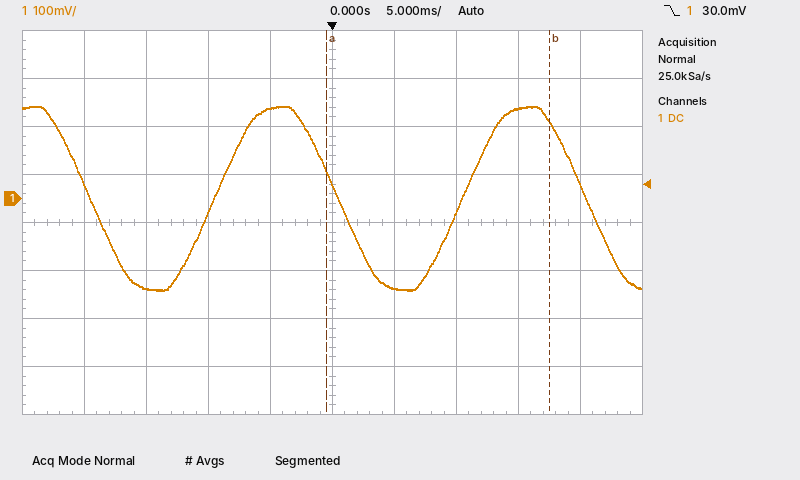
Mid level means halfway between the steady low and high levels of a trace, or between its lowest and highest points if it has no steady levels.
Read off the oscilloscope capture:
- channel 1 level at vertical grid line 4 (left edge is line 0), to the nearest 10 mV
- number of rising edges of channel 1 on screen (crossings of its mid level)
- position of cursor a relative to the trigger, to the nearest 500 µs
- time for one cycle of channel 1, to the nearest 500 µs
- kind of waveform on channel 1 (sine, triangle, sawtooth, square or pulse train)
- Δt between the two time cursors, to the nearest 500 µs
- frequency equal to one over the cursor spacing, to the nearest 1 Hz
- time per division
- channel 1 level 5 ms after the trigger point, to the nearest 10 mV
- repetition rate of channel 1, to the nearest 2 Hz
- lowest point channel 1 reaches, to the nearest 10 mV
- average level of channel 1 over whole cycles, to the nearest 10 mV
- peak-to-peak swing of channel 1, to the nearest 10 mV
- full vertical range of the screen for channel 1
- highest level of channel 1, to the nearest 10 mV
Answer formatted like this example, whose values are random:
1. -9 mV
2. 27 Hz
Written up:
1. 190 mV
2. 2
3. -500 µs
4. 20.0 ms
5. sine
6. 18.0 ms
7. 56 Hz
8. 5 ms
9. -190 mV
10. 50 Hz
11. -190 mV
12. 0 mV
13. 380 mV
14. 800 mV
15. 190 mV
